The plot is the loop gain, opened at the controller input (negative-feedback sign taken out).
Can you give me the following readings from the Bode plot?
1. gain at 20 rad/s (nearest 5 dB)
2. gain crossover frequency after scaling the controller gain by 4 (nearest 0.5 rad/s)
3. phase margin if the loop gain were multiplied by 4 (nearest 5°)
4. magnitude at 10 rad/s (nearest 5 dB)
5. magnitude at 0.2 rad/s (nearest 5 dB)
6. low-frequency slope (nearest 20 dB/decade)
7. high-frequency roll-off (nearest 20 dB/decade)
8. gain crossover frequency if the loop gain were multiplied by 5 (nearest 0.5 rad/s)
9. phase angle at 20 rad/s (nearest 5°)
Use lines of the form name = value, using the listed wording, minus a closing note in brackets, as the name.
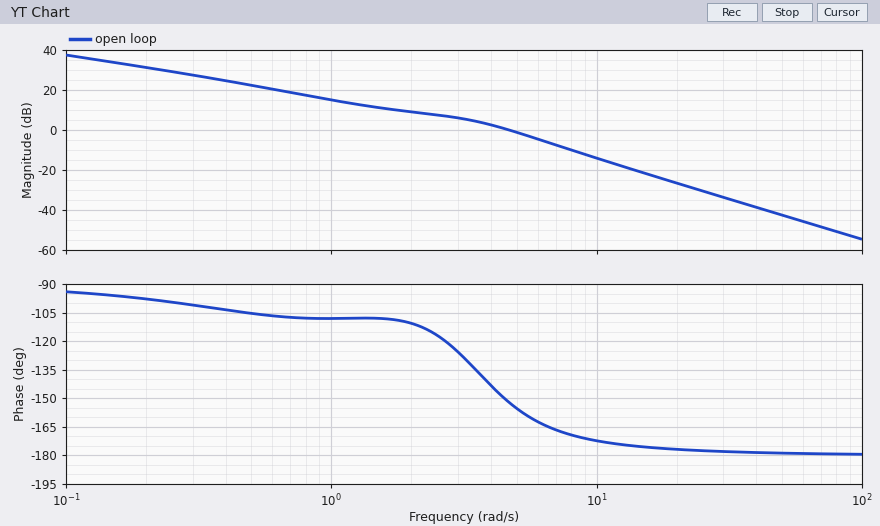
gain at 20 rad/s = -25 dB
gain crossover frequency after scaling the controller gain by 4 = 9.0 rad/s
phase margin if the loop gain were multiplied by 4 = 10°
magnitude at 10 rad/s = -15 dB
magnitude at 0.2 rad/s = 30 dB
low-frequency slope = -20 dB/decade
high-frequency roll-off = -40 dB/decade
gain crossover frequency if the loop gain were multiplied by 5 = 10.0 rad/s
phase angle at 20 rad/s = -175°
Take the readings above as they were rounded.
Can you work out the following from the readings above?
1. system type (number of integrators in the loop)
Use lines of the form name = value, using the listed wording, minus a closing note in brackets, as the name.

system type = 1
